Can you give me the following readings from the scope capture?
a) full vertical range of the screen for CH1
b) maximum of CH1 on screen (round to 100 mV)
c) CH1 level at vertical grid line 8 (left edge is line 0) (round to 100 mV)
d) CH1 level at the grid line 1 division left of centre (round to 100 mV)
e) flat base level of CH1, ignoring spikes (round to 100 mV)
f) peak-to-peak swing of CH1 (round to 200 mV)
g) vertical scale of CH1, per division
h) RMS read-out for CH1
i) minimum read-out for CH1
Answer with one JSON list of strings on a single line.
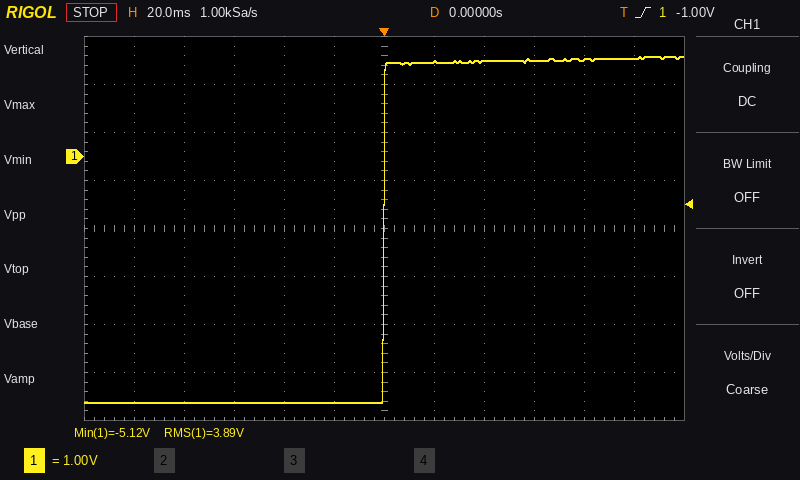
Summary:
["8 V", "2.1 V", "2.0 V", "-5.1 V", "-5.1 V", "7.2 V", "1 V", "3.89 V", "-5.12 V"]
